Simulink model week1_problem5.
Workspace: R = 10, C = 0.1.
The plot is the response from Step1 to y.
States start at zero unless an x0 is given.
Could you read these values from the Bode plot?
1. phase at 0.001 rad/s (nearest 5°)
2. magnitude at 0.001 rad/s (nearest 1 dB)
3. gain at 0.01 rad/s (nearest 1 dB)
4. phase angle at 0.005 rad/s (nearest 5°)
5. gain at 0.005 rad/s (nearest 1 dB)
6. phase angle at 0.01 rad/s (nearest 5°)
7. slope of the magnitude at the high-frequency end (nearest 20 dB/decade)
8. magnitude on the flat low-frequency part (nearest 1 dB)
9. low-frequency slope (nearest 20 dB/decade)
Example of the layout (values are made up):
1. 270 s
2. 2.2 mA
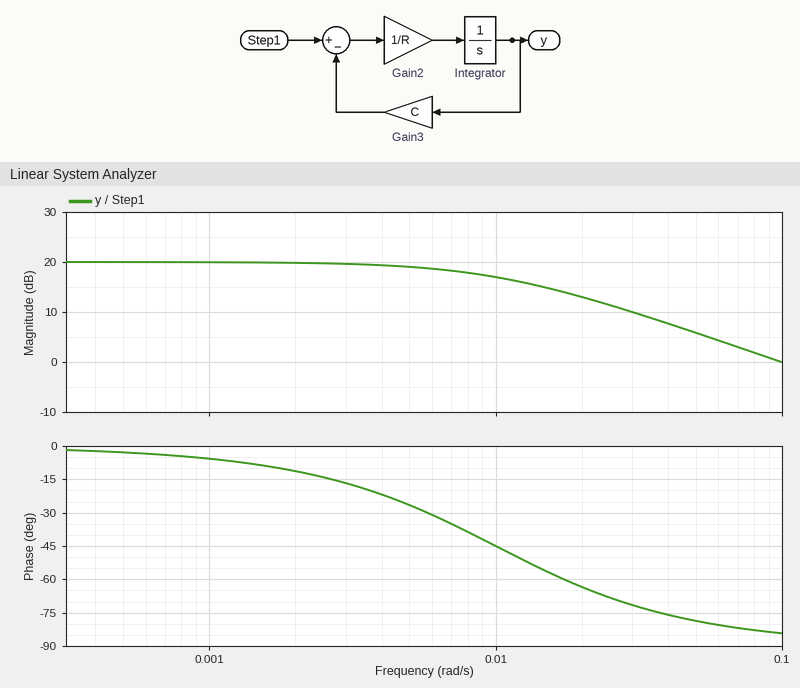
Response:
1. -5°
2. 20 dB
3. 17 dB
4. -25°
5. 19 dB
6. -45°
7. -20 dB/decade
8. 20 dB
9. 0 dB/decade
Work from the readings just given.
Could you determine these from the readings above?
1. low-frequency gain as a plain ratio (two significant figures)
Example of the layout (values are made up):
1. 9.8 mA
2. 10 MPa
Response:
1. 10
